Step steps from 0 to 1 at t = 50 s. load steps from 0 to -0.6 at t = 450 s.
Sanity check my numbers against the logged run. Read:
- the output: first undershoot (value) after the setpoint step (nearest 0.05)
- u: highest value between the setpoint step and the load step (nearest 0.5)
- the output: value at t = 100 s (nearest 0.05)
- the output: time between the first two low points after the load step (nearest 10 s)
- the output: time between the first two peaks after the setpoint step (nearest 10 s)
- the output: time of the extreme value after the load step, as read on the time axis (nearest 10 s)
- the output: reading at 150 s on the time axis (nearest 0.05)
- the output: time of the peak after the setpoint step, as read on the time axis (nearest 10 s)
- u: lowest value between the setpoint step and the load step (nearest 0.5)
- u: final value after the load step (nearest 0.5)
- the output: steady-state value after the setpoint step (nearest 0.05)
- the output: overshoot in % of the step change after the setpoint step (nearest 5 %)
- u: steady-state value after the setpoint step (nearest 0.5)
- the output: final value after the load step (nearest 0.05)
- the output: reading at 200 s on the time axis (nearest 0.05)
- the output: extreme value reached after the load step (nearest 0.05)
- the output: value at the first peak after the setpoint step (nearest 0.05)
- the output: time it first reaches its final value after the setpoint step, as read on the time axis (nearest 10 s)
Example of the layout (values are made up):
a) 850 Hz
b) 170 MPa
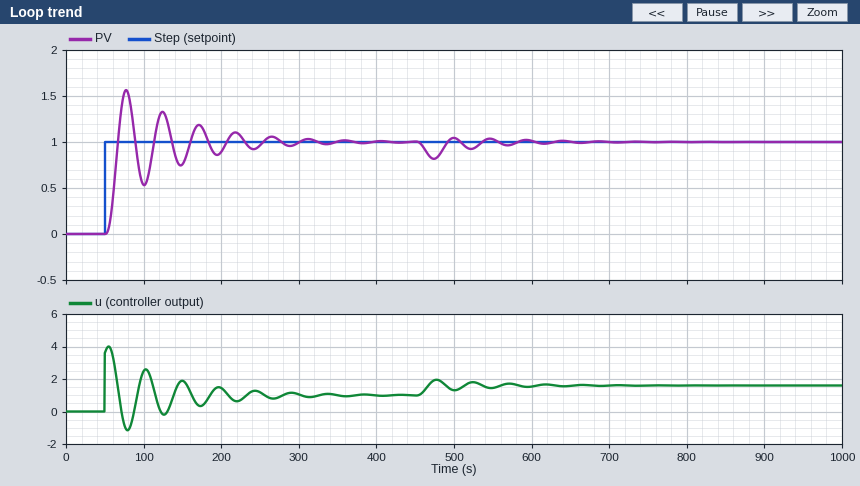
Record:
a) 0.55
b) 4.0
c) 0.55
d) 50 s
e) 50 s
f) 470 s
g) 0.75
h) 80 s
i) -1.0
j) 1.5
k) 1.00
l) 55 %
m) 1.0
n) 1.00
o) 0.90
p) 0.80
q) 1.55
r) 70 s
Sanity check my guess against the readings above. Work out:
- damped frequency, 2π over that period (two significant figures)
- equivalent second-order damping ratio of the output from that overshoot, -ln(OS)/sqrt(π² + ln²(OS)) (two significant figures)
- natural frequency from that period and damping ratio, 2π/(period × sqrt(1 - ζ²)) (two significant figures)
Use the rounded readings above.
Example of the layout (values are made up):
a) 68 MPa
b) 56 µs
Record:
a) 0.13 rad/s
b) 0.19
c) 0.13 rad/s
